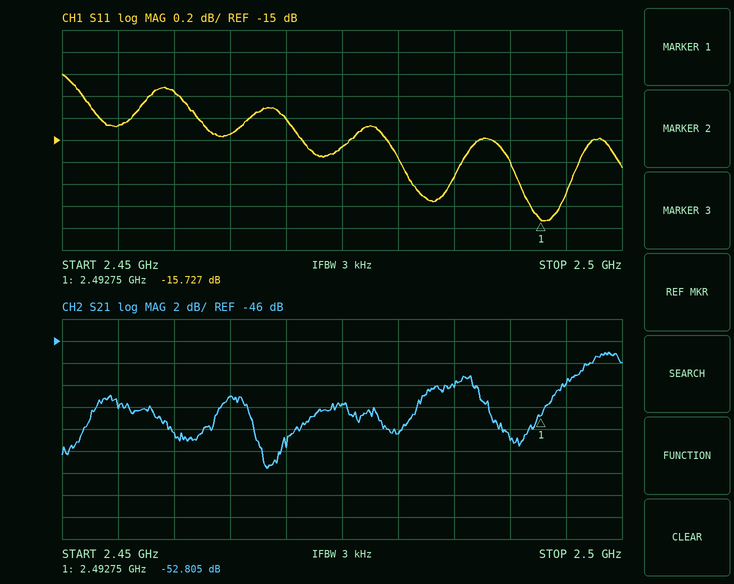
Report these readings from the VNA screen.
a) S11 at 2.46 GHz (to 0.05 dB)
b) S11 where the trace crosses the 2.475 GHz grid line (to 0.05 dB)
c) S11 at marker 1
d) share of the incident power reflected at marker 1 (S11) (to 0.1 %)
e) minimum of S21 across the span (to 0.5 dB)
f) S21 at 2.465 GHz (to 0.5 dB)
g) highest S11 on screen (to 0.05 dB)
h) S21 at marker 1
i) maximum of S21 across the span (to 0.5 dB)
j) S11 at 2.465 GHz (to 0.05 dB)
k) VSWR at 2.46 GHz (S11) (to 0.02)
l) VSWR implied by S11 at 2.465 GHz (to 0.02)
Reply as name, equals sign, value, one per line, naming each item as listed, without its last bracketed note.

S11 at 2.46 GHz = -14.55 dB
S11 where the trace crosses the 2.475 GHz grid line = -15.05 dB
S11 at marker 1 = -15.727 dB
share of the incident power reflected at marker 1 (S11) = 2.7 %
minimum of S21 across the span = -57.5 dB
S21 at 2.465 GHz = -51.0 dB
highest S11 on screen = -14.40 dB
S21 at marker 1 = -52.805 dB
maximum of S21 across the span = -47.0 dB
S11 at 2.465 GHz = -14.95 dB
VSWR at 2.46 GHz (S11) = 1.46
VSWR implied by S11 at 2.465 GHz = 1.44
